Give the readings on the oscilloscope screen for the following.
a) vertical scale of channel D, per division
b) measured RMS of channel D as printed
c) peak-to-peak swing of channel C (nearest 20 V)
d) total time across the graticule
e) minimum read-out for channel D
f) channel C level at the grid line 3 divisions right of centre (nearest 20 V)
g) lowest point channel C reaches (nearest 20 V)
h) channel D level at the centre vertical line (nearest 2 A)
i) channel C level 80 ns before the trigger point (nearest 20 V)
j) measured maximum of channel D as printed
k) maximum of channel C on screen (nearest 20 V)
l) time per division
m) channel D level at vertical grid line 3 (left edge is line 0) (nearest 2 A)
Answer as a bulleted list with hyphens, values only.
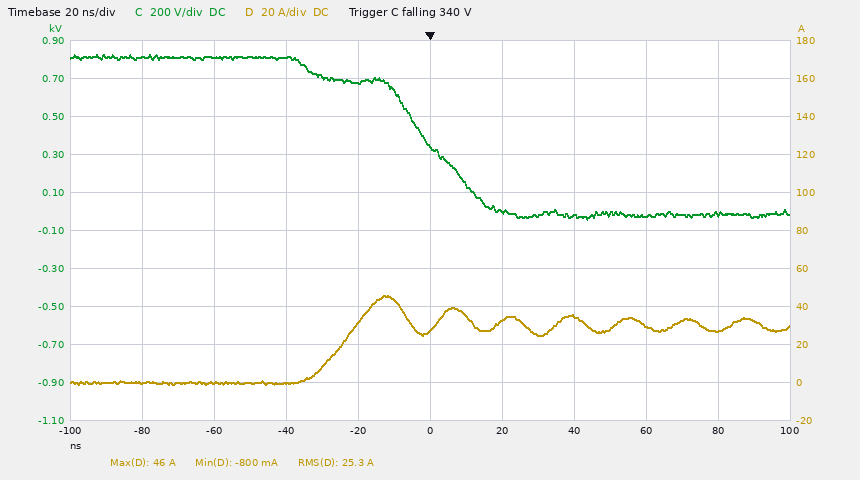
- 20 A
- 25.3 A
- 860 V
- 200 ns
- -800 mA
- -20 V
- -40 V
- 28 A
- 820 V
- 46 A
- 820 V
- 20 ns
- 0 A
